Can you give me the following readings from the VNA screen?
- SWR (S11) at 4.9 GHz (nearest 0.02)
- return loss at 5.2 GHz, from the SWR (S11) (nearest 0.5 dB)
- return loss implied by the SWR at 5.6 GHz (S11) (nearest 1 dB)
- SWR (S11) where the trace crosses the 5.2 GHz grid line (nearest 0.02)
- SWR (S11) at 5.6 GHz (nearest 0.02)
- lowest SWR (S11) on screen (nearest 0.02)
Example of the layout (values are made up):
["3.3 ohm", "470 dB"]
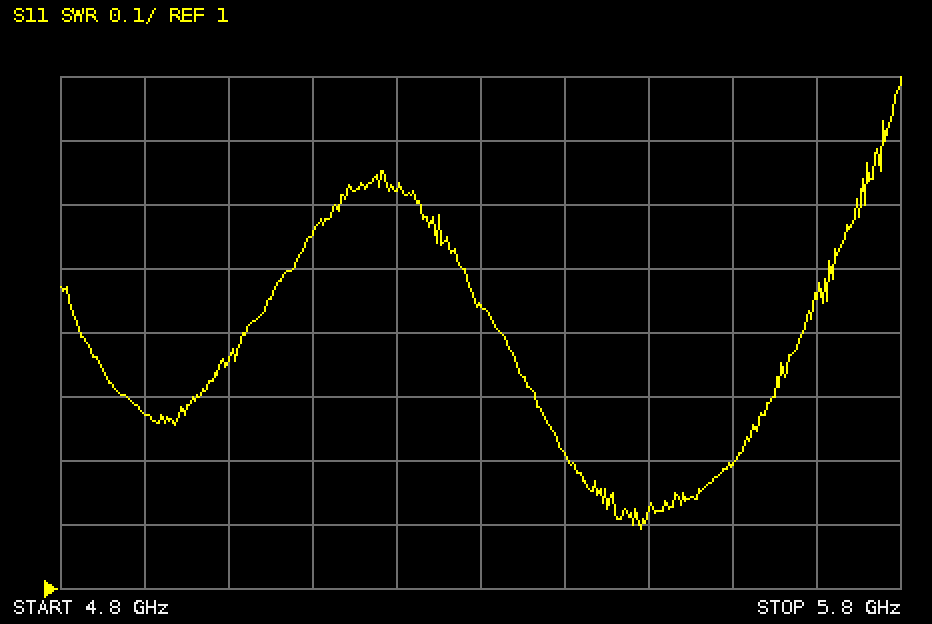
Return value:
["1.28", "12.5 dB", "21 dB", "1.62", "1.20", "1.10"]
